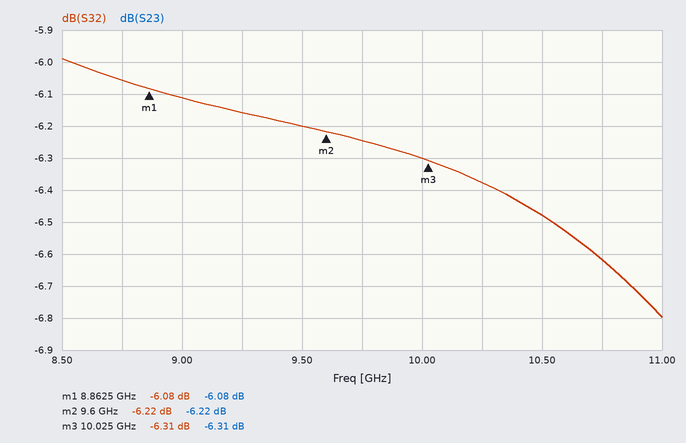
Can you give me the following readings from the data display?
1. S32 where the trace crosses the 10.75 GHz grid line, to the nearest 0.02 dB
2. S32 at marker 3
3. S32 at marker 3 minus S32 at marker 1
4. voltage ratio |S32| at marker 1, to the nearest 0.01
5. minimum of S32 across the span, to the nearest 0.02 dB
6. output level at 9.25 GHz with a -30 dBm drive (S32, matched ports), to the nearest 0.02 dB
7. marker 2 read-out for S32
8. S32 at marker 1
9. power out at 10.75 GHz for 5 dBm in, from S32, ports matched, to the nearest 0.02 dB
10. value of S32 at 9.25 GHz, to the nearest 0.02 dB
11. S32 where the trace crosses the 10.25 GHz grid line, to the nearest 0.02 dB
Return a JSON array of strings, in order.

["-6.62 dB", "-6.31 dB", "-0.23 dB", "0.50", "-6.80 dB", "-36.16 dBm", "-6.22 dB", "-6.08 dB", "-1.62 dBm", "-6.16 dB", "-6.38 dB"]
